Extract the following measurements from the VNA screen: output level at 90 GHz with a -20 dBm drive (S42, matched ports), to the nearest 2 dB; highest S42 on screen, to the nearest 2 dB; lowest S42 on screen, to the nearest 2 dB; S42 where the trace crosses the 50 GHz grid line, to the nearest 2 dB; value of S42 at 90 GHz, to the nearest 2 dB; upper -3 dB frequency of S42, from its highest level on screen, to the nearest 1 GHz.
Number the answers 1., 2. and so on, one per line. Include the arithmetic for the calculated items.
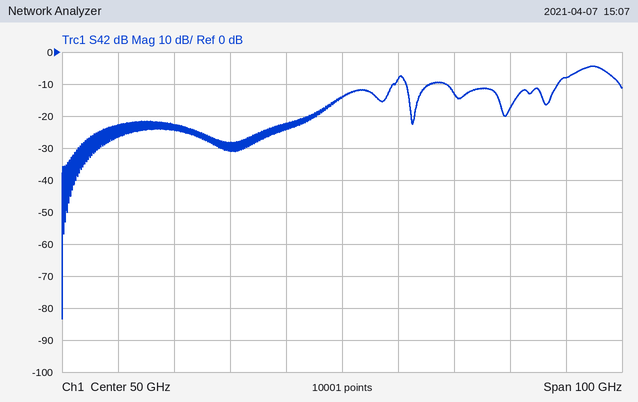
1. -20 dBm + (-8 dB) = -28 dBm
2. -4 dB
3. -84 dB
4. -14 dB
5. -8 dB
6. 98 GHz
